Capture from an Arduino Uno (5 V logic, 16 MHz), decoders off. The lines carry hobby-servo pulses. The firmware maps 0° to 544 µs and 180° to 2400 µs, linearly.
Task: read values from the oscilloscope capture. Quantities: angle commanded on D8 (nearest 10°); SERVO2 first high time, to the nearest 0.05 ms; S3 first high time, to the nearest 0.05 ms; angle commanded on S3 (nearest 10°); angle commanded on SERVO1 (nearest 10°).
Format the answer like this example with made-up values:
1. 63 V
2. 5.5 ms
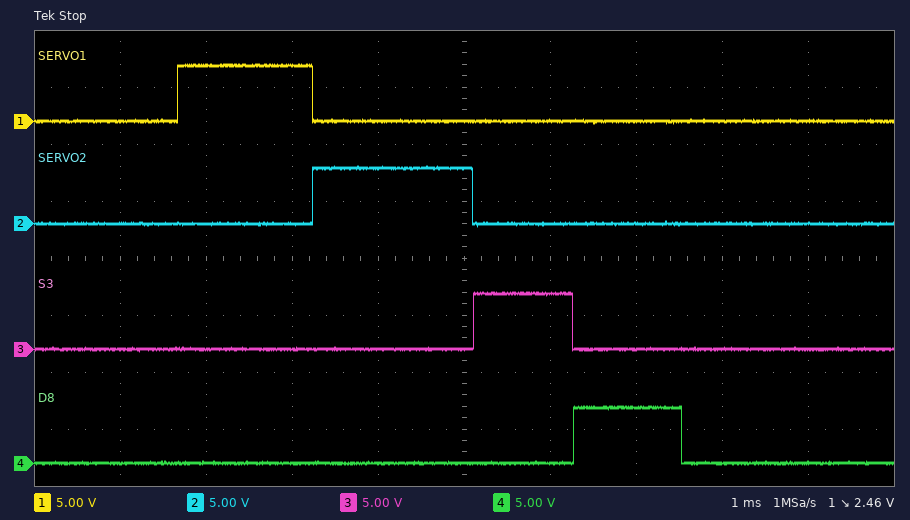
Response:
1. 70°
2. 1.85 ms
3. 1.15 ms
4. 60°
5. 100°
